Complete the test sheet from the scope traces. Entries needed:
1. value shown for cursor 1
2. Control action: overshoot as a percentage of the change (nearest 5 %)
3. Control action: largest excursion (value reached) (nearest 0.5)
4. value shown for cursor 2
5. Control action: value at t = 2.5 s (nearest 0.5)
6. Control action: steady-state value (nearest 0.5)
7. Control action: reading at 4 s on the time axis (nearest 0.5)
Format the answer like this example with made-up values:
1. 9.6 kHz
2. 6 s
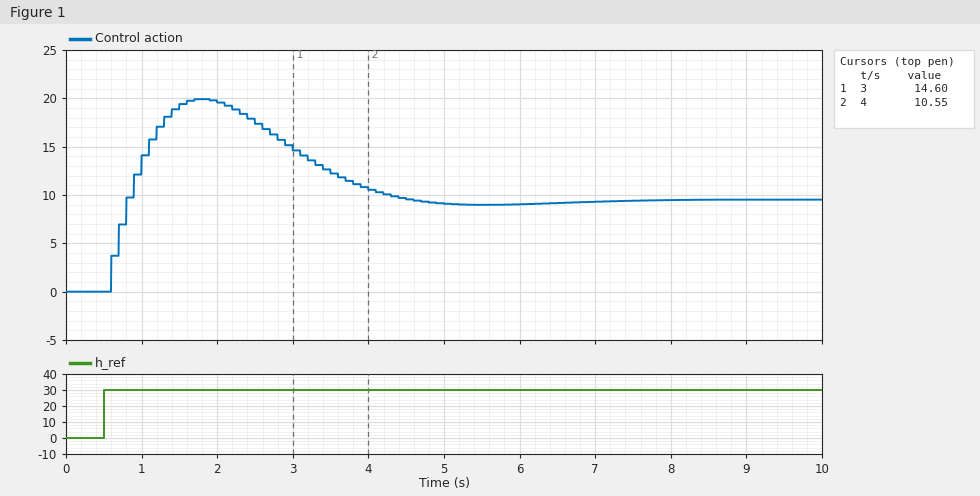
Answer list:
1. 14.60
2. 110 %
3. 20.0
4. 10.55
5. 17.5
6. 9.5
7. 10.5
